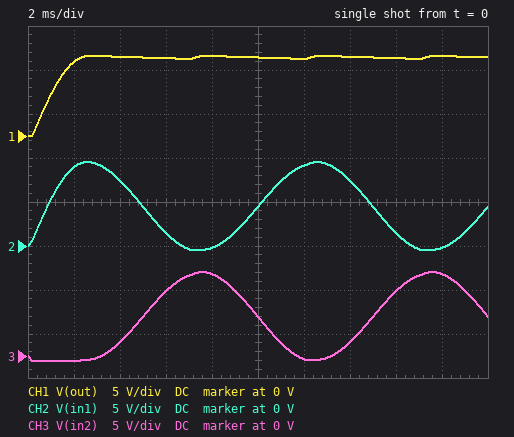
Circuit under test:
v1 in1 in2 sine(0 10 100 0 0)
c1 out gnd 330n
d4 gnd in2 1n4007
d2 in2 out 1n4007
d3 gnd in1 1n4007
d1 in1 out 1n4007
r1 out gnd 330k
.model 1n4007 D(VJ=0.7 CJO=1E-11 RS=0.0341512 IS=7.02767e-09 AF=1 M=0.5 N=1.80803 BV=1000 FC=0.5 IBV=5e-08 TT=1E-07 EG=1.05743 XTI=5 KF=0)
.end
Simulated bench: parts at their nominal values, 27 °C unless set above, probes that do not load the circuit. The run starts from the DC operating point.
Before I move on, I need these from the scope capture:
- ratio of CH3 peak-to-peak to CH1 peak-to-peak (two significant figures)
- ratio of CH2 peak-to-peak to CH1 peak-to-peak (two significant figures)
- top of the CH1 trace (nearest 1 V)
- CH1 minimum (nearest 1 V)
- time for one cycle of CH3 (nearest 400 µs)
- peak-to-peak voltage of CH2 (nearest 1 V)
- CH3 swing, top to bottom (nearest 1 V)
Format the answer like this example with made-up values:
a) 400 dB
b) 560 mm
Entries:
a) 1.1
b) 1.1
c) 9 V
d) 0 V
e) 10.0 ms
f) 10 V
g) 10 V
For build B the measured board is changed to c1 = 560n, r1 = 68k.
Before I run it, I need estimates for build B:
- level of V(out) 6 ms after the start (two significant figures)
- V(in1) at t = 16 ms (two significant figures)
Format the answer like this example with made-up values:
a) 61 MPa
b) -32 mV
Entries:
a) 8.3 V
b) 1.2 V
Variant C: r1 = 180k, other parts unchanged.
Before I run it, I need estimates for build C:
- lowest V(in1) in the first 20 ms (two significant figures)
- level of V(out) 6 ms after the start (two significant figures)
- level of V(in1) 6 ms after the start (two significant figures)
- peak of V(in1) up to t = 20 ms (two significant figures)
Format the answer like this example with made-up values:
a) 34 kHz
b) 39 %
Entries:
a) -530 mV
b) 8.6 V
c) 1.4 V
d) 9.5 V
